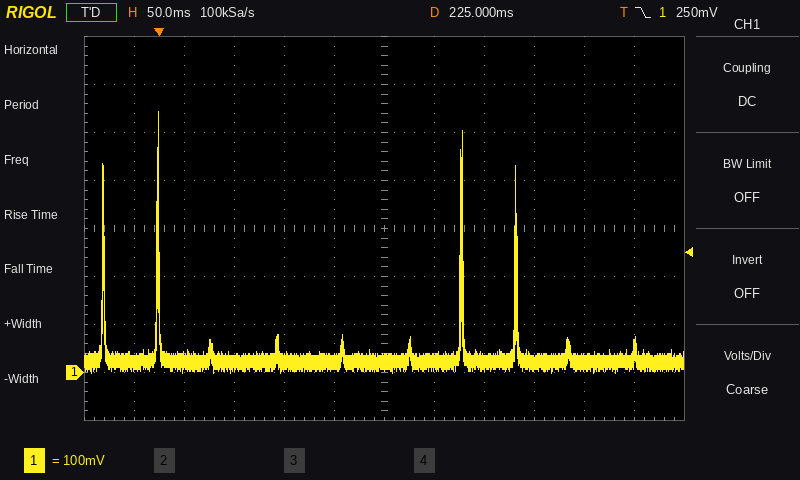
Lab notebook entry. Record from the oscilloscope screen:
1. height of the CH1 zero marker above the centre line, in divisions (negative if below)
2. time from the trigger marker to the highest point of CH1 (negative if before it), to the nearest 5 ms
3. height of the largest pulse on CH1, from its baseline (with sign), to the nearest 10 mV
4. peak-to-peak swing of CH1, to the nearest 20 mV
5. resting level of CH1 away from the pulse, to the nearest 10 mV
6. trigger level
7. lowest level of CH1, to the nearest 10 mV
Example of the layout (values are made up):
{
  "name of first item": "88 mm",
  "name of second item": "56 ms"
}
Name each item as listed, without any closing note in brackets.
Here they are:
{
  "height of the CH1 zero marker above the centre line, in divisions": "-3.0 div",
  "time from the trigger marker to the highest point of CH1 (negative if before it), to the nearest 5 ms": "0 ms",
  "height of the largest pulse on CH1, from its baseline (with sign), to the nearest 10 mV": "+520 mV",
  "peak-to-peak swing of CH1, to the nearest 20 mV": "540 mV",
  "resting level of CH1 away from the pulse, to the nearest 10 mV": "20 mV",
  "trigger level": "250 mV",
  "lowest level of CH1, to the nearest 10 mV": "0 mV"
}
